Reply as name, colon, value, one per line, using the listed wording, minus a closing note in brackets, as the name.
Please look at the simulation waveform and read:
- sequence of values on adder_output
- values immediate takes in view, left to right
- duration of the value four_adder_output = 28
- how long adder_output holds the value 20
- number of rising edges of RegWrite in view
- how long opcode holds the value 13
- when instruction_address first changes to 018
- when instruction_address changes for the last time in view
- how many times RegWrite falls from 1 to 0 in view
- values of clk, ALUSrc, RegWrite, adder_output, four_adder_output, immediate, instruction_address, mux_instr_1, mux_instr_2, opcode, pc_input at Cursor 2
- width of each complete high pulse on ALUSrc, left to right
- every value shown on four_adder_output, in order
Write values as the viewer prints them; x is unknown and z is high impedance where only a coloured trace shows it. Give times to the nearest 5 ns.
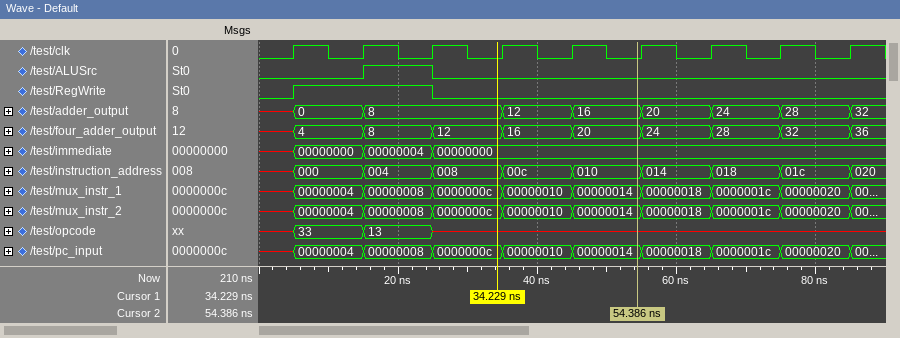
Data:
sequence of values on adder_output: x, 0, 8, 12, 16, 20, 24, 28, 32
values immediate takes in view, left to right: x, 00000000, 00000004, 00000000
duration of the value four_adder_output = 28: 10 ns
how long adder_output holds the value 20: 10 ns
number of rising edges of RegWrite in view: 1
how long opcode holds the value 13: 10 ns
when instruction_address first changes to 018: 65 ns
when instruction_address changes for the last time in view: 85 ns
how many times RegWrite falls from 1 to 0 in view: 1
values of clk, ALUSrc, RegWrite, adder_output, four_adder_output, immediate, instruction_address, mux_instr_1, mux_instr_2, opcode, pc_input at Cursor 2: clk=0, ALUSrc=0, RegWrite=0, adder_output=16, four_adder_output=20, immediate=00000000, instruction_address=010, mux_instr_1=00000014, mux_instr_2=00000014, opcode=x, pc_input=00000014
width of each complete high pulse on ALUSrc, left to right: 10 ns
every value shown on four_adder_output, in order: x, 4, 8, 12, 16, 20, 24, 28, 32, 36
